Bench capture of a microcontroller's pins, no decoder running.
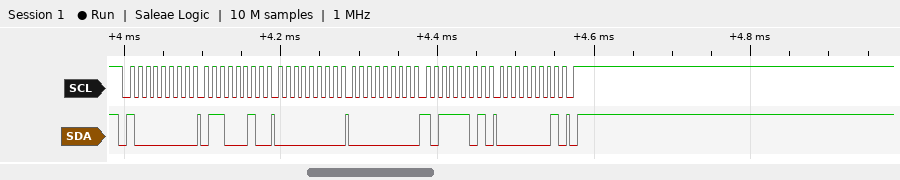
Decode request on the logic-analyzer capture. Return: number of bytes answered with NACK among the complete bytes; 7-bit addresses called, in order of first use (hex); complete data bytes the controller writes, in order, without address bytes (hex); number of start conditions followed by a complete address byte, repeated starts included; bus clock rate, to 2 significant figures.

0
0x40
62 00 00 BD 01
1
100 kHz
